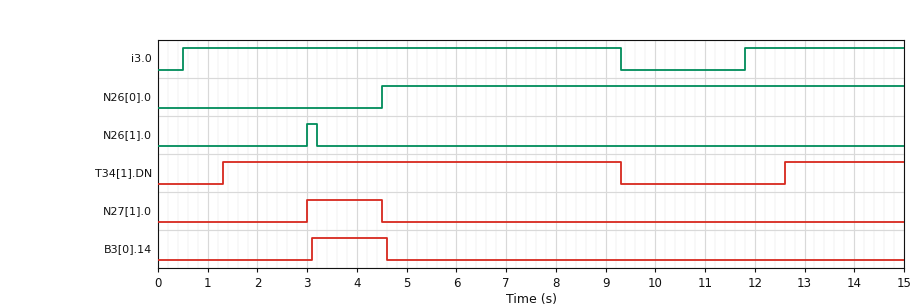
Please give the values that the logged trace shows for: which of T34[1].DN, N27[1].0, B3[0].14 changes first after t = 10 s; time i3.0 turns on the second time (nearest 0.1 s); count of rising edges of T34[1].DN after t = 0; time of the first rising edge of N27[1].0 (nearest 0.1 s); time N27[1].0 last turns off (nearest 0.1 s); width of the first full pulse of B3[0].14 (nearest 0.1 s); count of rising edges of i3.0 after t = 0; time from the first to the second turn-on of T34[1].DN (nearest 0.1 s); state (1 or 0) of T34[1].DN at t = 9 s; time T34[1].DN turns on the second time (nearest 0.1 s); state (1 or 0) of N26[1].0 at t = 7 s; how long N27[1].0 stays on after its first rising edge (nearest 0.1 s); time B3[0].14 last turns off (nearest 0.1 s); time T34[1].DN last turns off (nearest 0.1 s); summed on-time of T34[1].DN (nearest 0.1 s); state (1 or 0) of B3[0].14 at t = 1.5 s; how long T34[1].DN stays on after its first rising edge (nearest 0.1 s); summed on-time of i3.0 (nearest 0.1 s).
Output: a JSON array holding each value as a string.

["T34[1].DN", "11.8 s", "2", "3.0 s", "4.5 s", "1.5 s", "2", "11.3 s", "1", "12.6 s", "0", "1.5 s", "4.6 s", "9.3 s", "10.4 s", "0", "8.0 s", "12.0 s"]
